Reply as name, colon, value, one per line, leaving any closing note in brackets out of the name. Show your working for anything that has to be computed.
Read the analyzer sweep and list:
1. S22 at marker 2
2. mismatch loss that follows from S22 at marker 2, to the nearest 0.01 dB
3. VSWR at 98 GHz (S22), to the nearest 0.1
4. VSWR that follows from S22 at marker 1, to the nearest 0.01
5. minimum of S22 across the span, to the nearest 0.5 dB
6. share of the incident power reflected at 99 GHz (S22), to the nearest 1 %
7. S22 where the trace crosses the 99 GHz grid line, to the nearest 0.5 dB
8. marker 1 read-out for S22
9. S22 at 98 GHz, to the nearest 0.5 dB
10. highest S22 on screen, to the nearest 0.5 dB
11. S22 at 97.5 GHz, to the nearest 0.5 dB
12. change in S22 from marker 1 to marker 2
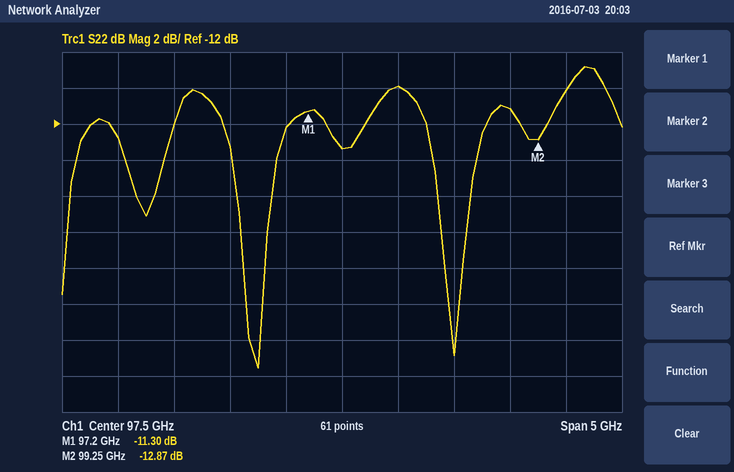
S22 at marker 2: -12.87 dB
mismatch loss that follows from S22 at marker 2, to the nearest 0.01 dB: −10 log10(1 − 10^(-12.87/10)) ≈ 0.23 dB
VSWR at 98 GHz (S22), to the nearest 0.1: |Γ| = 10^(-10/20) = 0.3162; VSWR = (1 + 0.3162)/(1 − 0.3162) ≈ 1.9
VSWR that follows from S22 at marker 1, to the nearest 0.01: (1 + 0.2723)/(1 − 0.2723) ≈ 1.75
minimum of S22 across the span, to the nearest 0.5 dB: -25.5 dB
share of the incident power reflected at 99 GHz (S22), to the nearest 1 %: 10^(-11/10) ≈ 8 %
S22 where the trace crosses the 99 GHz grid line, to the nearest 0.5 dB: -11.0 dB
marker 1 read-out for S22: -11.30 dB
S22 at 98 GHz, to the nearest 0.5 dB: -10.0 dB
highest S22 on screen, to the nearest 0.5 dB: -9.0 dB
S22 at 97.5 GHz, to the nearest 0.5 dB: -13.5 dB
change in S22 from marker 1 to marker 2: -12.87 − (-11.3) = -1.57 dB
